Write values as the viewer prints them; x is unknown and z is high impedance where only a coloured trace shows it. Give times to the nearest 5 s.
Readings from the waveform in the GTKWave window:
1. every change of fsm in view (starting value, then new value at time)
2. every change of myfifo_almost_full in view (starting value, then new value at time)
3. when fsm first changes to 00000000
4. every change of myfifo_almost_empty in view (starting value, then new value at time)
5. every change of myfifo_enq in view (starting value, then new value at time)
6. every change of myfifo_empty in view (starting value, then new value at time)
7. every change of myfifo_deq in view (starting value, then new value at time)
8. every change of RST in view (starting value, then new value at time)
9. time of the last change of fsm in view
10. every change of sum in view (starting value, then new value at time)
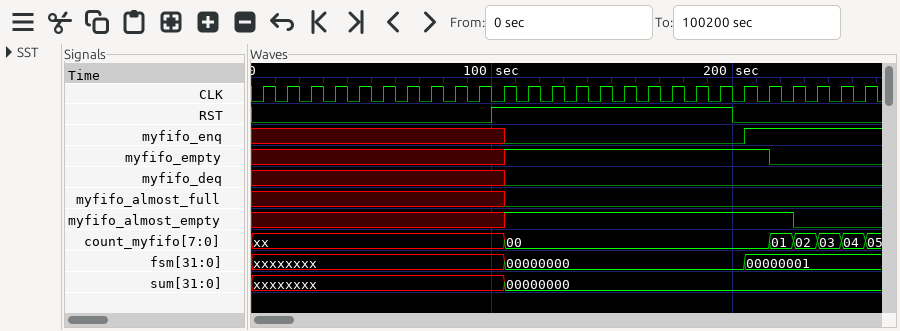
xxxxxxxx, 00000000 at 105 s, 00000001 at 205 s
x, 0 at 105 s
105 s
x, 1 at 105 s, 0 at 225 s
x, 0 at 105 s, 1 at 205 s
x, 1 at 105 s, 0 at 215 s
x, 0 at 105 s
0, 1 at 100 s, 0 at 200 s
205 s
xxxxxxxx, 00000000 at 105 s
